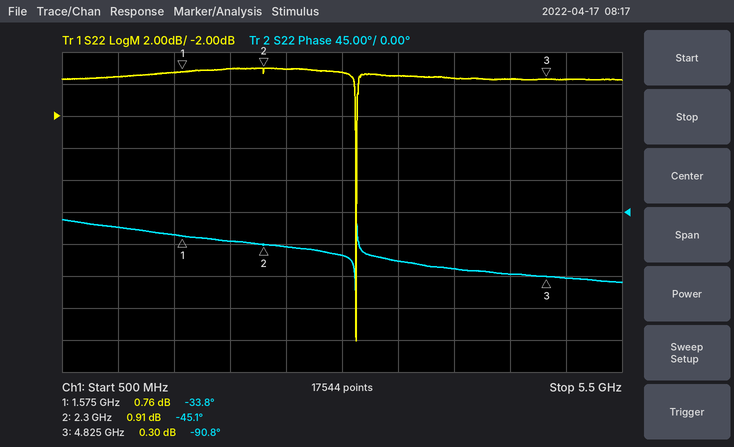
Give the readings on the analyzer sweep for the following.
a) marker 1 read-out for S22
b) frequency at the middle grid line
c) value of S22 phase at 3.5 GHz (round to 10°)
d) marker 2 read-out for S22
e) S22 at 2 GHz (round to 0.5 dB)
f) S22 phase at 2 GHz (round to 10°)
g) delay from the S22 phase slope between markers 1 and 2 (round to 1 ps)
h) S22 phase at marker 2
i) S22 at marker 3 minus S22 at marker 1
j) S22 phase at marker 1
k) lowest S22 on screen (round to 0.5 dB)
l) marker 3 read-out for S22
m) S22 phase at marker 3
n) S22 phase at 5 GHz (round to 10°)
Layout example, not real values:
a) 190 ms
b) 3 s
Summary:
a) 0.76 dB
b) 3 GHz
c) -70°
d) 0.91 dB
e) 1.0 dB
f) -40°
g) 43 ps
h) -45.1°
i) -0.46 dB
j) -33.8°
k) -16.0 dB
l) 0.30 dB
m) -90.8°
n) -90°
